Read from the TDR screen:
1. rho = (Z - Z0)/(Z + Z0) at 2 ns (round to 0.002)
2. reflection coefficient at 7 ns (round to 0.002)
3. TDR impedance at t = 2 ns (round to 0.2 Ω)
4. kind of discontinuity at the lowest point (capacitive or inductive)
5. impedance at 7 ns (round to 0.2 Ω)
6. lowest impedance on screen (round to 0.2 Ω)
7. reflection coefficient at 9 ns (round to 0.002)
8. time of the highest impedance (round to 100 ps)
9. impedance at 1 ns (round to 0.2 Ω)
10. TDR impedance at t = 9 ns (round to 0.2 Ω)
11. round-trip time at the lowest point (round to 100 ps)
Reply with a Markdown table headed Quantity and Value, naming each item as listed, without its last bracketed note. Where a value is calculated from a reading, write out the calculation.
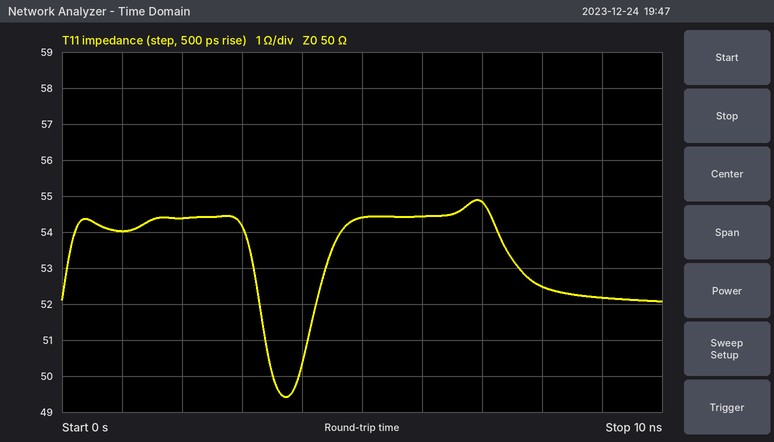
| Quantity | Value |
|---|---|
| rho = (Z - Z0)/(Z + Z0) at 2 ns | (54.4 − 50)/(54.4 + 50) ≈ +0.042 |
| reflection coefficient at 7 ns | (54.8 − 50)/(54.8 + 50) ≈ +0.046 |
| TDR impedance at t = 2 ns | 54.4 Ω |
| kind of discontinuity at the lowest point | capacitive |
| impedance at 7 ns | 54.8 Ω |
| lowest impedance on screen | 49.4 Ω |
| reflection coefficient at 9 ns | (52.2 − 50)/(52.2 + 50) ≈ +0.022 |
| time of the highest impedance | 6.9 ns |
| impedance at 1 ns | 54.0 Ω |
| TDR impedance at t = 9 ns | 52.2 Ω |
| round-trip time at the lowest point | 3.7 ns |
